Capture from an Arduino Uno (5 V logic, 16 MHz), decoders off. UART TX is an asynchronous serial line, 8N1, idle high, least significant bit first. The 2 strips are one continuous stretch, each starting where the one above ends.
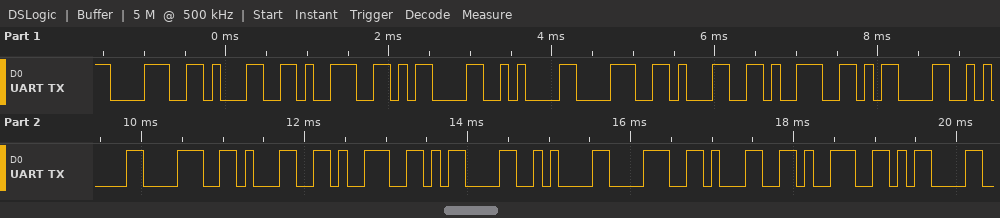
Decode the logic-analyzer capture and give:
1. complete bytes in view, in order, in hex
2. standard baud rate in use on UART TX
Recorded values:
38 31 39 0D 0A 38 31 39 0D 0A 38 31 39 0D 0A 38 31 39 0D
9600 baud
